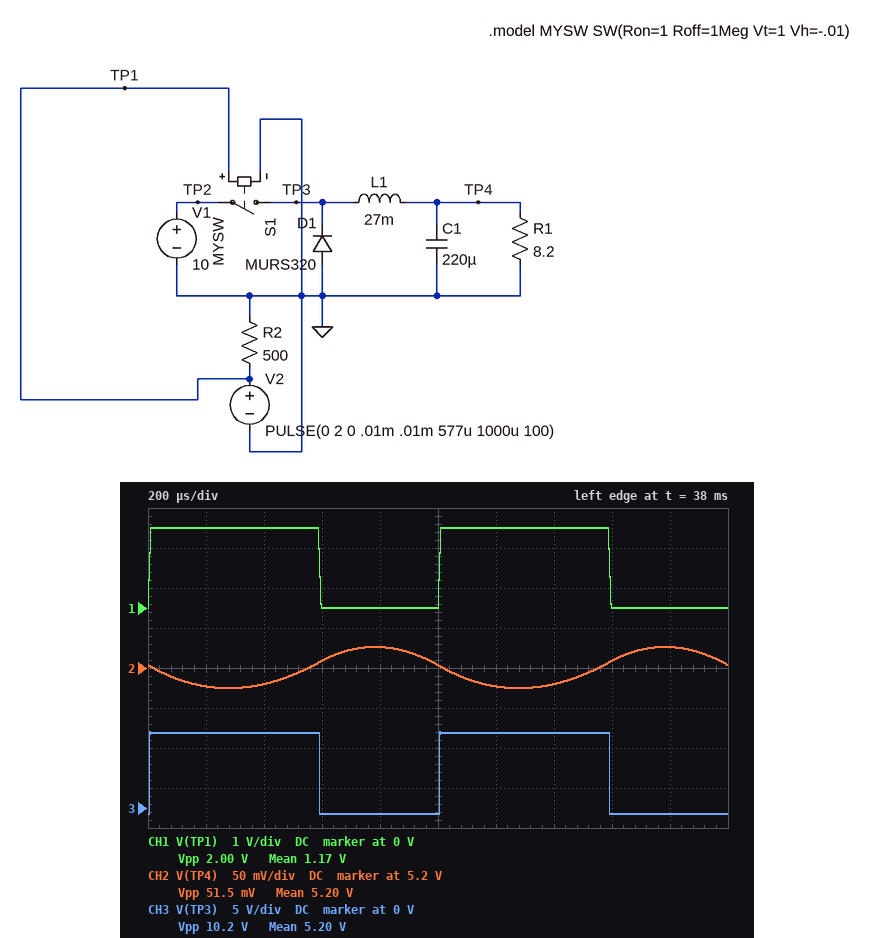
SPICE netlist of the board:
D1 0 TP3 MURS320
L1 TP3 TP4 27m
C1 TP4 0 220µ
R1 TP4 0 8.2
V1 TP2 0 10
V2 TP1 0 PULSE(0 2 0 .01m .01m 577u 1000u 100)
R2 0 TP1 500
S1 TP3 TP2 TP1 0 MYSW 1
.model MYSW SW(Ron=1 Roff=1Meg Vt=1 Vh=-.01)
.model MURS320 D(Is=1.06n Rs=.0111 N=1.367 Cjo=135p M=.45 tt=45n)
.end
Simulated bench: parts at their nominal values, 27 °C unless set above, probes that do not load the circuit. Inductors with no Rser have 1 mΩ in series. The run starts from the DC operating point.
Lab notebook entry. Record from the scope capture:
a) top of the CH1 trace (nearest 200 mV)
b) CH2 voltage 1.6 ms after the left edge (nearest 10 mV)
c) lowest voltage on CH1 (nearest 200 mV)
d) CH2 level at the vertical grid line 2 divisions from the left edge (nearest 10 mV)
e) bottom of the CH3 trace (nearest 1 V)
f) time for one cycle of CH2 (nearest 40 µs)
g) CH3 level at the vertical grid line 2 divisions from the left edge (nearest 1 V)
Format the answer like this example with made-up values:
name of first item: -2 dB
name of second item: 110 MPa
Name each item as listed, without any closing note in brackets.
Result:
top of the CH1 trace: 2.0 V
CH2 voltage 1.6 ms after the left edge: 5.21 V
lowest voltage on CH1: 0 V
CH2 level at the vertical grid line 2 divisions from the left edge: 5.18 V
bottom of the CH3 trace: -1 V
time for one cycle of CH2: 1.00 ms
CH3 level at the vertical grid line 2 divisions from the left edge: 9 V
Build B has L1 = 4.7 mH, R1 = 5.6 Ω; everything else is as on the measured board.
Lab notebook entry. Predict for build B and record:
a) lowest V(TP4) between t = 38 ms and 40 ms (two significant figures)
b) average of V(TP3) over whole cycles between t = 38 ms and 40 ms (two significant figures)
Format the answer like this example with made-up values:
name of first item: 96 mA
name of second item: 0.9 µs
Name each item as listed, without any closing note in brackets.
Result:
lowest V(TP4) between t = 38 ms and 40 ms: 4.9 V
average of V(TP3) over whole cycles between t = 38 ms and 40 ms: 5.0 V
